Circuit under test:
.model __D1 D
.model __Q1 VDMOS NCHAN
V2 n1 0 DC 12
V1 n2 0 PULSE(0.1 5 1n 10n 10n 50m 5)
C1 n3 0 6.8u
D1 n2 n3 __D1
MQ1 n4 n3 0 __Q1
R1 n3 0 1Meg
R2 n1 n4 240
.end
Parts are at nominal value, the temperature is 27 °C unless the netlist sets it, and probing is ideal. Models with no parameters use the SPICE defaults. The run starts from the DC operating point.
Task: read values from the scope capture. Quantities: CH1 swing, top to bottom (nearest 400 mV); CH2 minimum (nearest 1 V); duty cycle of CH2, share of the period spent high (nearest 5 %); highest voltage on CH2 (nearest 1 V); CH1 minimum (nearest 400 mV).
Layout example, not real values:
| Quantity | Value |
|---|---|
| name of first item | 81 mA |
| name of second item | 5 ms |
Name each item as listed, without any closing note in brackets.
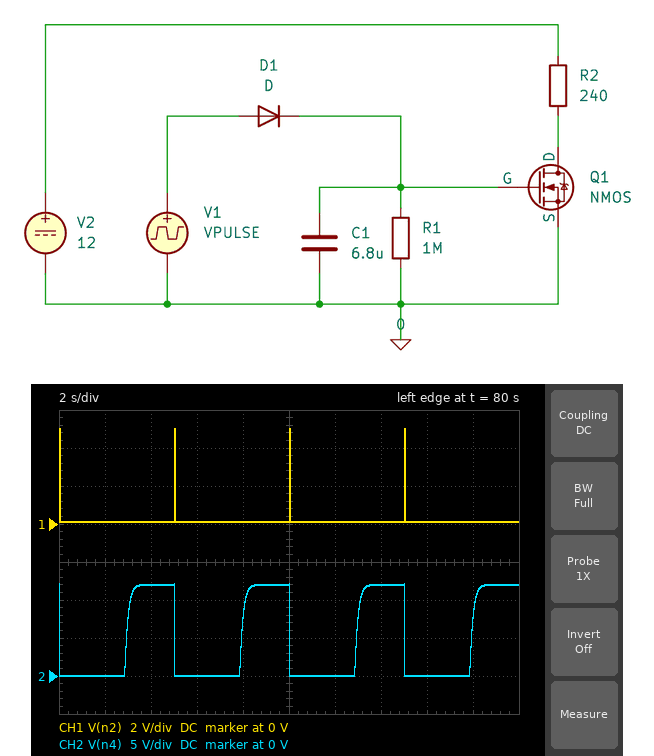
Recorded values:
| Quantity | Value |
|---|---|
| CH1 swing, top to bottom | 4.8 V |
| CH2 minimum | 0 V |
| duty cycle of CH2, share of the period spent high | 40 % |
| highest voltage on CH2 | 12 V |
| CH1 minimum | 0 V |
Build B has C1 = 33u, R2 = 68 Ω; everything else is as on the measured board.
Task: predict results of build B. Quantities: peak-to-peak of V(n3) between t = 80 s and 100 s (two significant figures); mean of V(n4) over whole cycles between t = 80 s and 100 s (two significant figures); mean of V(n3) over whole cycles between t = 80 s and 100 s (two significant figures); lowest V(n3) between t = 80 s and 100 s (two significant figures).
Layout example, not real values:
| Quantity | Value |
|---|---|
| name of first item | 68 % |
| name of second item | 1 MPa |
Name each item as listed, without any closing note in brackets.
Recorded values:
| Quantity | Value |
|---|---|
| peak-to-peak of V(n3) between t = 80 s and 100 s | 620 mV |
| mean of V(n4) over whole cycles between t = 80 s and 100 s | 4.6 mV |
| mean of V(n3) over whole cycles between t = 80 s and 100 s | 4.1 V |
| lowest V(n3) between t = 80 s and 100 s | 3.8 V |
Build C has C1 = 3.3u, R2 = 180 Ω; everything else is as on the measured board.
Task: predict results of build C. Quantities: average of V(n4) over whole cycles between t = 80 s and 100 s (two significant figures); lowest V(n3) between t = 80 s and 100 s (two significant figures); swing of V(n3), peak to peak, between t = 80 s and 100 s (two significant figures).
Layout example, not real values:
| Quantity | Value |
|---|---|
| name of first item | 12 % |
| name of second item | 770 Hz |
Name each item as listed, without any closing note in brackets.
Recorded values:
| Quantity | Value |
|---|---|
| average of V(n4) over whole cycles between t = 80 s and 100 s | 8.5 V |
| lowest V(n3) between t = 80 s and 100 s | 1.0 V |
| swing of V(n3), peak to peak, between t = 80 s and 100 s | 3.5 V |
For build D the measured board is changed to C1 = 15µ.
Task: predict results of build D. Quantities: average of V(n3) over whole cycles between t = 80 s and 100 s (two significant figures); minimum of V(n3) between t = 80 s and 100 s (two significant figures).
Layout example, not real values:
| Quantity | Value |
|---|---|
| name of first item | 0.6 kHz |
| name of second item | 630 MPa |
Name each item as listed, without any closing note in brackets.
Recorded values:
| Quantity | Value |
|---|---|
| average of V(n3) over whole cycles between t = 80 s and 100 s | 3.8 V |
| minimum of V(n3) between t = 80 s and 100 s | 3.2 V |
